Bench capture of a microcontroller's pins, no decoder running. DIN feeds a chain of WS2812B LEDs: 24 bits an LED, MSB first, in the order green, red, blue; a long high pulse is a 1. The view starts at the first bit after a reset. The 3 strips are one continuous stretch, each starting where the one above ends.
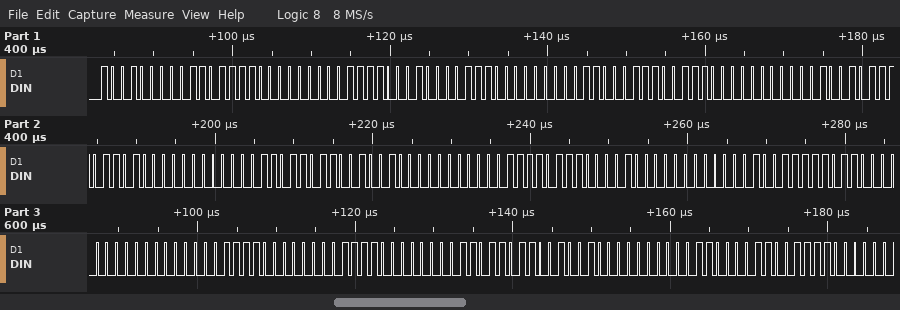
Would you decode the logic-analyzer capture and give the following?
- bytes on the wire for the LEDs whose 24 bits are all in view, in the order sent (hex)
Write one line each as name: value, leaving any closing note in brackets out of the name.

bytes on the wire for the LEDs whose 24 bits are all in view, in the order sent: 90 6F 00 78 87 00 63 9C 00 4B B4 00 36 C9 00 1E E1 00 09 F6 00 00 F0 0F 00 DB 24 00 C3 3C
